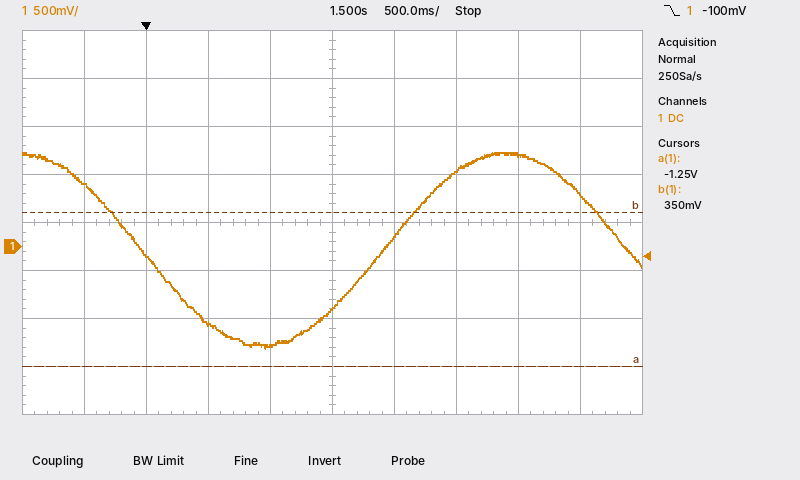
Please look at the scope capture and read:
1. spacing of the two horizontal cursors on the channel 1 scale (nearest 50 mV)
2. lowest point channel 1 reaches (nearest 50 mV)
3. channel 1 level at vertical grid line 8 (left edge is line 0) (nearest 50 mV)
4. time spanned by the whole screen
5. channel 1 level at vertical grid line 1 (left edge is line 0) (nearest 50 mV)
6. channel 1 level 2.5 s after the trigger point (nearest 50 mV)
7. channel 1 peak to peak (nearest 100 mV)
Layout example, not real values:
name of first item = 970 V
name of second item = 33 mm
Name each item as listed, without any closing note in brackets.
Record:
spacing of the two horizontal cursors on the channel 1 scale = 1.60 V
lowest point channel 1 reaches = -1.05 V
channel 1 level at vertical grid line 8 (left edge is line 0) = 950 mV
time spanned by the whole screen = 5 s
channel 1 level at vertical grid line 1 (left edge is line 0) = 650 mV
channel 1 level 2.5 s after the trigger point = 800 mV
channel 1 peak to peak = 2.00 V
